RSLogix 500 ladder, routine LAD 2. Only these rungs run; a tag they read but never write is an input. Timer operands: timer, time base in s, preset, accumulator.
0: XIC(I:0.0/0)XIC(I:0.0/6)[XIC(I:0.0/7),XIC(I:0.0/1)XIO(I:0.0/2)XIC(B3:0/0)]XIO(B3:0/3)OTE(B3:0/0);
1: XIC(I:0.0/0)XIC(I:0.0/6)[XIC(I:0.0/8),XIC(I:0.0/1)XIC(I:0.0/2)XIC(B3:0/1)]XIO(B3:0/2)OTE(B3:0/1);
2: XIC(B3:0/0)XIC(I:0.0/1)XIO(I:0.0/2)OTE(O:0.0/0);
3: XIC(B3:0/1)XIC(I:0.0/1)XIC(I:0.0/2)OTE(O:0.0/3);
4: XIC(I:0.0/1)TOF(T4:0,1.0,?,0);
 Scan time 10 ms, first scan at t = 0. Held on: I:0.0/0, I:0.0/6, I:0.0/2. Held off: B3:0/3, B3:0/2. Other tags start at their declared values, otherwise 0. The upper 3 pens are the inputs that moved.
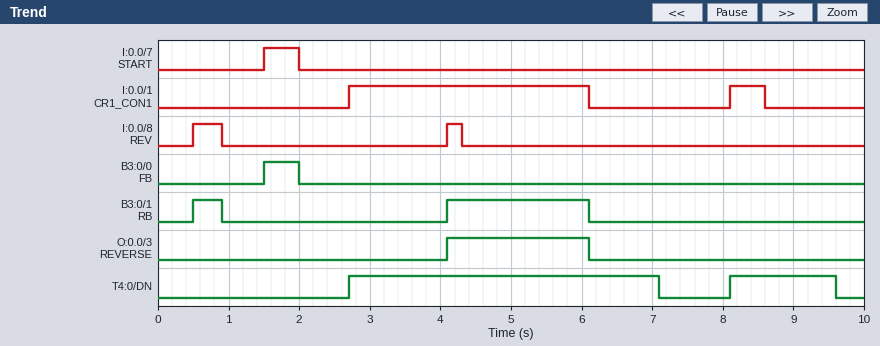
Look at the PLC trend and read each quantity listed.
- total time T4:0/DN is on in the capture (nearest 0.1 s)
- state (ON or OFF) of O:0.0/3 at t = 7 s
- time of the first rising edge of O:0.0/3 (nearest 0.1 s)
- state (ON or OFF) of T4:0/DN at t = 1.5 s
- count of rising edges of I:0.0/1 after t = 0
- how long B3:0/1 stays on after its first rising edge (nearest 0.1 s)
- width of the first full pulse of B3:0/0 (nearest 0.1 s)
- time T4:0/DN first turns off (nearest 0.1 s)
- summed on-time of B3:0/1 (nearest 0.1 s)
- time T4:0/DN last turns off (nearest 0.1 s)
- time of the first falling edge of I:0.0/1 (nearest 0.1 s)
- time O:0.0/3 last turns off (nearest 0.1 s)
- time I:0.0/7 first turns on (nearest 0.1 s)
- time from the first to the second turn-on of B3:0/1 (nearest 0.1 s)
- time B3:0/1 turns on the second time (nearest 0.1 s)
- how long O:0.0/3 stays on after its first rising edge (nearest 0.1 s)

5.9 s
OFF
4.1 s
OFF
2
0.4 s
0.5 s
7.1 s
2.4 s
9.6 s
6.1 s
6.1 s
1.5 s
3.6 s
4.1 s
2.0 s
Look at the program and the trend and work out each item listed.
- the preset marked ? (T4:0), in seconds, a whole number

1 s
